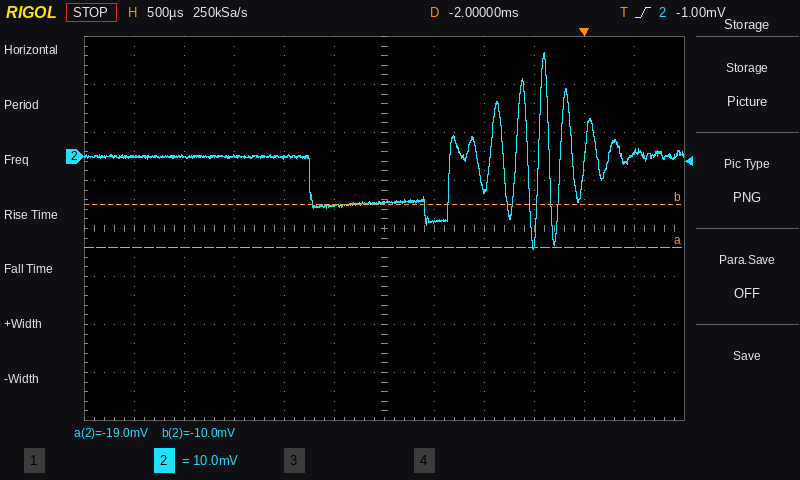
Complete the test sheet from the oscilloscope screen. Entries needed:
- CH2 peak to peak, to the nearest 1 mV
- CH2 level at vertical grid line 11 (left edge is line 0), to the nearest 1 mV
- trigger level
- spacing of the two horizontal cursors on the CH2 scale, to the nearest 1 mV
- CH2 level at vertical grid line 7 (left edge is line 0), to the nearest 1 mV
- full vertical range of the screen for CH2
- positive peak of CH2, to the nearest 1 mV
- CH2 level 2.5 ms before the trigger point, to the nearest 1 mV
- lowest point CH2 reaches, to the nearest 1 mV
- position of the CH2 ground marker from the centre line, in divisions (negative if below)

41 mV
1 mV
-1.00 mV
9 mV
-14 mV
80 mV
22 mV
-10 mV
-19 mV
+1.5 div
